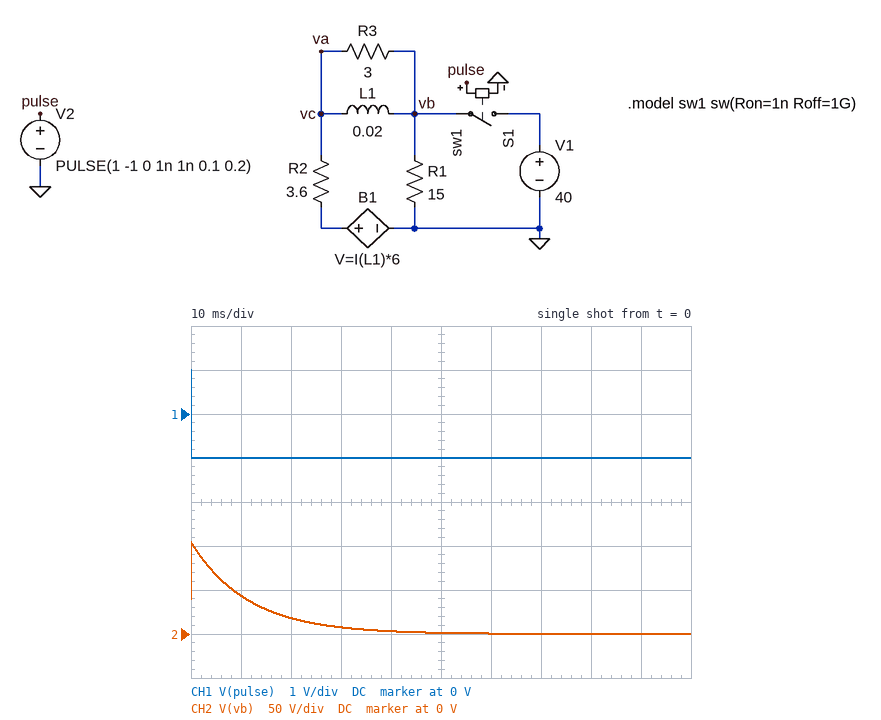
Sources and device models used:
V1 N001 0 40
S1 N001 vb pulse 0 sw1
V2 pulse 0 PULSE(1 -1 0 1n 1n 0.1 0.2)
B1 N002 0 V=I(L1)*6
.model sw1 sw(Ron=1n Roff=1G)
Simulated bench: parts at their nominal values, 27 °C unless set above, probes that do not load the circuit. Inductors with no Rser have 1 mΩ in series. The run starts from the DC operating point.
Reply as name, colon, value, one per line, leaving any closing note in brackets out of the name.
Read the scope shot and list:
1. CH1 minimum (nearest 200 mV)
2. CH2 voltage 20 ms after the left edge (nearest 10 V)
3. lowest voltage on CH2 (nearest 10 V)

CH1 minimum: -1.0 V
CH2 voltage 20 ms after the left edge: 20 V
lowest voltage on CH2: 0 V
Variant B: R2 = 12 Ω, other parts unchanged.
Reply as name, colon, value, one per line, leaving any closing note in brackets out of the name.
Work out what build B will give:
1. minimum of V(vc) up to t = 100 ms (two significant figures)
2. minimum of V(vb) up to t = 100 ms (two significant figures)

minimum of V(vc) up to t = 100 ms: -16 V
minimum of V(vb) up to t = 100 ms: -30 V
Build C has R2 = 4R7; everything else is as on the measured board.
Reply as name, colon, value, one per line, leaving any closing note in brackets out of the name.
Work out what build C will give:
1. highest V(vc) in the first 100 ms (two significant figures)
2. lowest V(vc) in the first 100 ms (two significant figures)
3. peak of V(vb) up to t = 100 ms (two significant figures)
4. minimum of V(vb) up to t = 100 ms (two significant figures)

highest V(vc) in the first 100 ms: 130 V
lowest V(vc) in the first 100 ms: 15 mV
peak of V(vb) up to t = 100 ms: 180 V
minimum of V(vb) up to t = 100 ms: 21 mV
